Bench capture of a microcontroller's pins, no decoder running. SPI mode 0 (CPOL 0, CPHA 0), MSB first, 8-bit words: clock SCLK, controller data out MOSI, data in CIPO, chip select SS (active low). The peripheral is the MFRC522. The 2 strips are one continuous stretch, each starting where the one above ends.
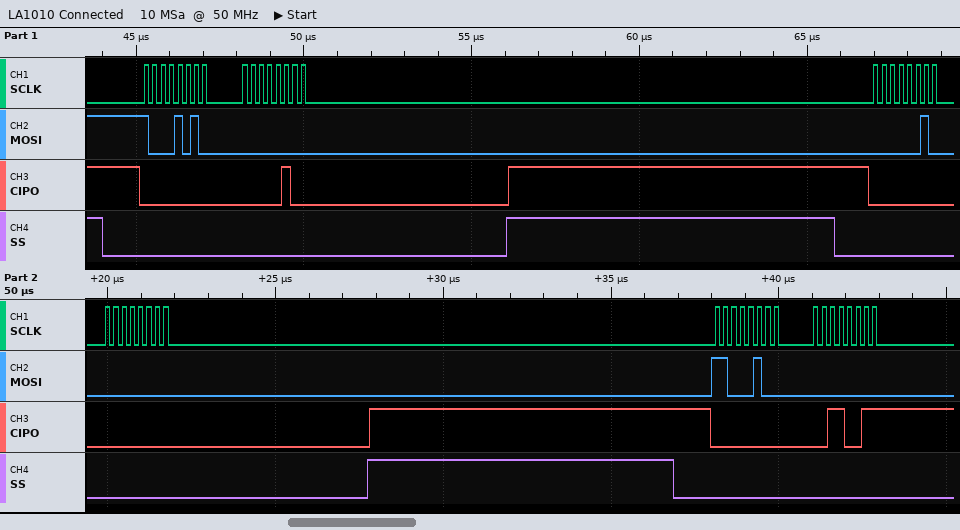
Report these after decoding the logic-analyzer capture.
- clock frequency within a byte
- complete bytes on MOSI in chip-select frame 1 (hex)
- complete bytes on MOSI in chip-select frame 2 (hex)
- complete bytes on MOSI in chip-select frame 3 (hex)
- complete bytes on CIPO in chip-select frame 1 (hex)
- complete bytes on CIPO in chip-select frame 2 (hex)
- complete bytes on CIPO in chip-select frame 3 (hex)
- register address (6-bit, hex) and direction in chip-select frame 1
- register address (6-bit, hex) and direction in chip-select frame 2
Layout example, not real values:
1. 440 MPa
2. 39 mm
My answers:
1. 4 MHz
2. 8A 00
3. 02 00
4. C4 00
5. 00 04
6. 00 00
7. 00 33
8. 0x05 read
9. 0x01 write
